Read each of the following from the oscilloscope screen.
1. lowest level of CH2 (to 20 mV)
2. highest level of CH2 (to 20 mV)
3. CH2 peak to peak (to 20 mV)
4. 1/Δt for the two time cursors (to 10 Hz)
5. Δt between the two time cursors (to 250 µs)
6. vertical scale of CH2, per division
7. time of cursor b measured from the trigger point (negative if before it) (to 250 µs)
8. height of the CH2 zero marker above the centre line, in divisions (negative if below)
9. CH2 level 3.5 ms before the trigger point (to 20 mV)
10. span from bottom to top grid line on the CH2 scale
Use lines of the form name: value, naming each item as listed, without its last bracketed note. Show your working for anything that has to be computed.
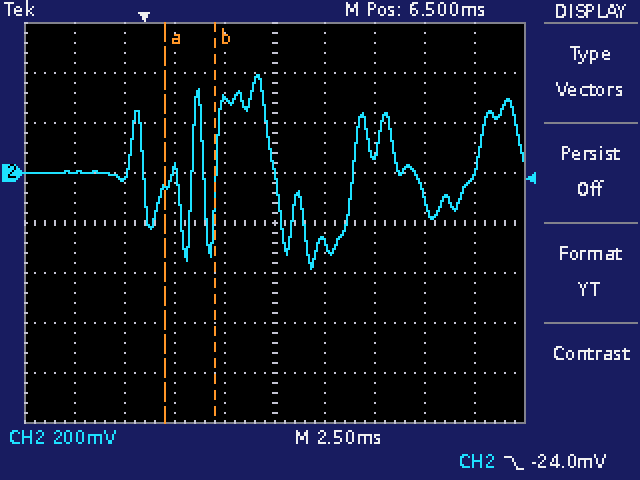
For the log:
lowest level of CH2: -380 mV
highest level of CH2: 400 mV
CH2 peak to peak: 400 mV − (-380 mV) = 780 mV
1/Δt for the two time cursors: 1 / 2.50 ms ≈ 400 Hz
Δt between the two time cursors: 2.50 ms
vertical scale of CH2, per division: 200 mV
time of cursor b measured from the trigger point (negative if before it): +3.50 ms
height of the CH2 zero marker above the centre line, in divisions: +1.0 div
CH2 level 3.5 ms before the trigger point: 0 mV
span from bottom to top grid line on the CH2 scale: 1.6 V
